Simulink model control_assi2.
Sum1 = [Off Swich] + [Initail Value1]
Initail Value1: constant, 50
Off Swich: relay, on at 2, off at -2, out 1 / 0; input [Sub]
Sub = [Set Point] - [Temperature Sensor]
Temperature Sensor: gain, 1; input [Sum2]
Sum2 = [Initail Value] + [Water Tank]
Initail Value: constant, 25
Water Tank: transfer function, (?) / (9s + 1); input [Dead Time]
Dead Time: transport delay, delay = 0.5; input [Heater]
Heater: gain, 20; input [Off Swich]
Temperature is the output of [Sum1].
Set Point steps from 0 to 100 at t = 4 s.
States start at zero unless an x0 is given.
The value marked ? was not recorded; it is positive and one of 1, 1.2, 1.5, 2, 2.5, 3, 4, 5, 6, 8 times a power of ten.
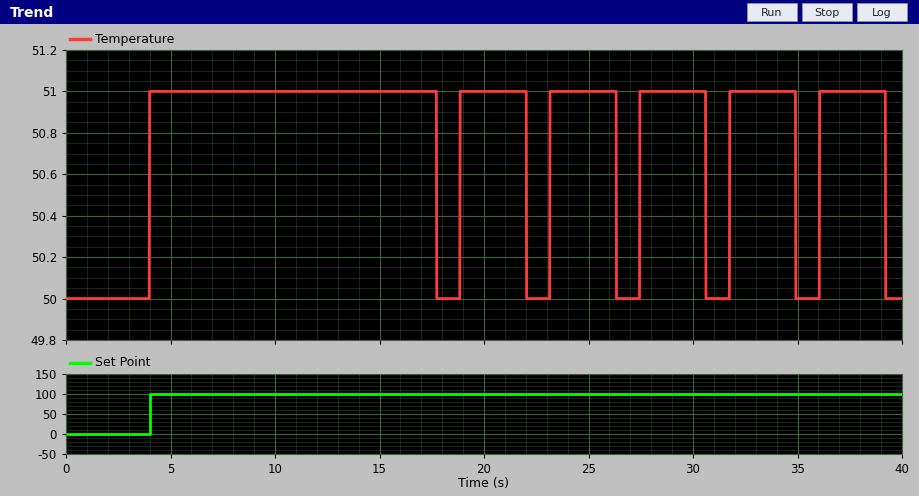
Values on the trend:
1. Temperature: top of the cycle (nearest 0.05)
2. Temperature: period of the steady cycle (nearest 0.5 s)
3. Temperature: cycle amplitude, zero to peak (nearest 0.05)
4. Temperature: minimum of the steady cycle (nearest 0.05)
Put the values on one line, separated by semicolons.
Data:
51.00; 4.5 s; 0.50; 50.00
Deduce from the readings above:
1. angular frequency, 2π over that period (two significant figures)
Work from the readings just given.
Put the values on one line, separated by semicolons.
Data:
1.4 rad/s
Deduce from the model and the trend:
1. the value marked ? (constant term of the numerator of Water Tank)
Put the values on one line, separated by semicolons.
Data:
5
